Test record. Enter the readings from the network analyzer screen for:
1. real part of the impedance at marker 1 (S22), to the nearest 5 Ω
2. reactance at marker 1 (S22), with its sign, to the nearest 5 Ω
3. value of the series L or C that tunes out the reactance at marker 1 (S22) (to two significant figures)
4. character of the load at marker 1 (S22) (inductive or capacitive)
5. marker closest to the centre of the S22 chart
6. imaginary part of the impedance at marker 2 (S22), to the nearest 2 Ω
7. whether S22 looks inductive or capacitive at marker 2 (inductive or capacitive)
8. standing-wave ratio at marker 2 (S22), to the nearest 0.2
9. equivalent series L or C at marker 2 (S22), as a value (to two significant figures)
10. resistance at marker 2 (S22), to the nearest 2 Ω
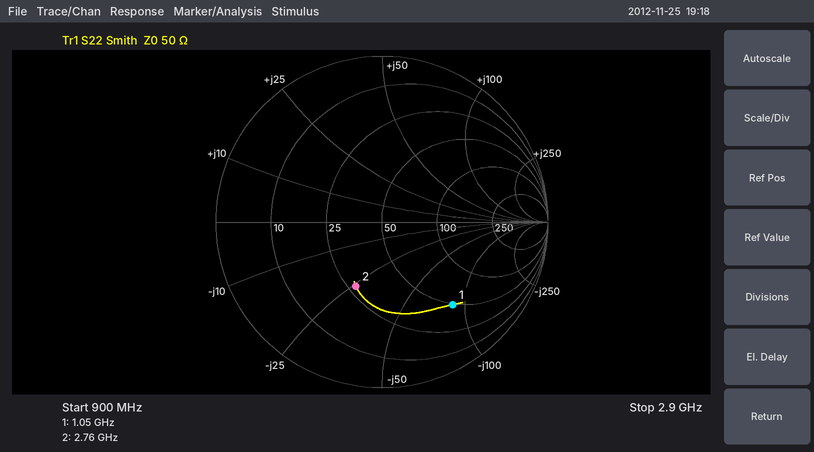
50 Ω
-85 Ω
13 nH
capacitive
marker 2
-26 Ω
capacitive
2.4
2.2 pF
28 Ω
